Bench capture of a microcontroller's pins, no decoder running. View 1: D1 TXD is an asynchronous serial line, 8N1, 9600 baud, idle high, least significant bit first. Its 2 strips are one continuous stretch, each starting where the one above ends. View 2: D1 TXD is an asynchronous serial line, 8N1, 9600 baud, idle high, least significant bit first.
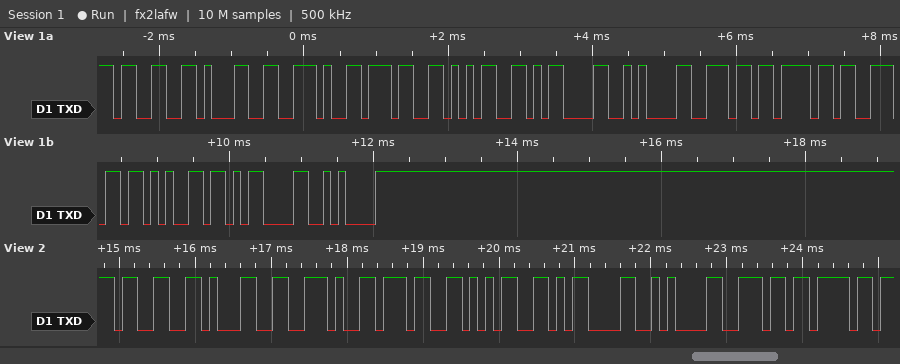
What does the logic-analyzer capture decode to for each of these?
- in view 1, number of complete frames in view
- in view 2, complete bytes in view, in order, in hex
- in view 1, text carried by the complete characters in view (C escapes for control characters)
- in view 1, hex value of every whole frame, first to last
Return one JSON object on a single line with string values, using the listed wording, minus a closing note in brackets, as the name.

{"in view 1, number of complete frames in view": "13", "in view 2, complete bytes in view, in order, in hex": "33 31 2E 37 35 0D 0A 6E 6F", "in view 1, text carried by the complete characters in view": "\"31.75\\r\\nnone\\r\\n\"", "in view 1, hex value of every whole frame, first to last": "33 31 2E 37 35 0D 0A 6E 6F 6E 65 0D 0A"}
